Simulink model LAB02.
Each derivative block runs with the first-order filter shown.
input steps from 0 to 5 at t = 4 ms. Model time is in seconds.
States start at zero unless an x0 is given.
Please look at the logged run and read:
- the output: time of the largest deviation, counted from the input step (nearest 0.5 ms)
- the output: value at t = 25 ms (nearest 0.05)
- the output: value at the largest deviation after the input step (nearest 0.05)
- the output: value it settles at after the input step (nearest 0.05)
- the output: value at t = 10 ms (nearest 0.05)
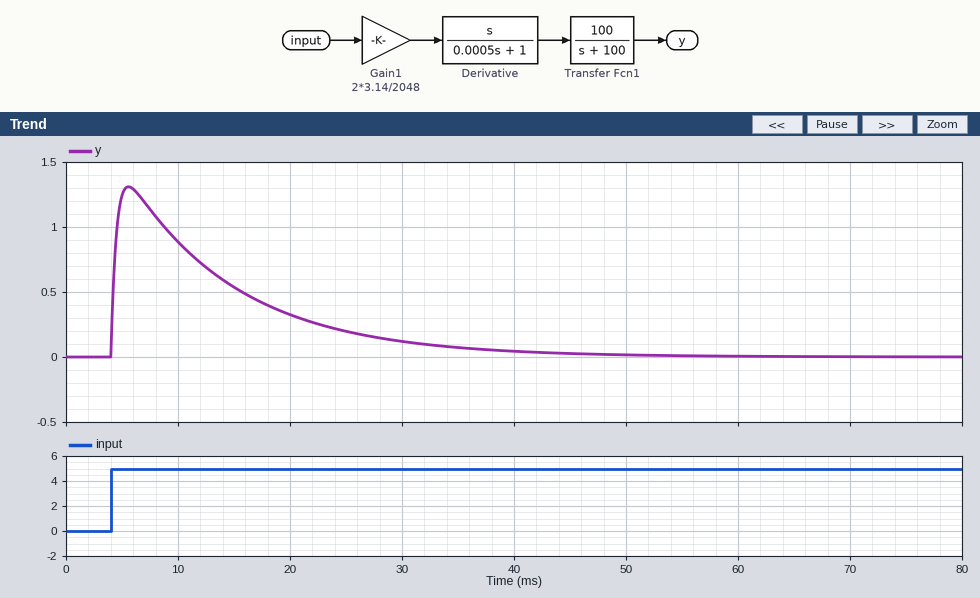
1.5 ms
0.20
1.30
0.00
0.90
